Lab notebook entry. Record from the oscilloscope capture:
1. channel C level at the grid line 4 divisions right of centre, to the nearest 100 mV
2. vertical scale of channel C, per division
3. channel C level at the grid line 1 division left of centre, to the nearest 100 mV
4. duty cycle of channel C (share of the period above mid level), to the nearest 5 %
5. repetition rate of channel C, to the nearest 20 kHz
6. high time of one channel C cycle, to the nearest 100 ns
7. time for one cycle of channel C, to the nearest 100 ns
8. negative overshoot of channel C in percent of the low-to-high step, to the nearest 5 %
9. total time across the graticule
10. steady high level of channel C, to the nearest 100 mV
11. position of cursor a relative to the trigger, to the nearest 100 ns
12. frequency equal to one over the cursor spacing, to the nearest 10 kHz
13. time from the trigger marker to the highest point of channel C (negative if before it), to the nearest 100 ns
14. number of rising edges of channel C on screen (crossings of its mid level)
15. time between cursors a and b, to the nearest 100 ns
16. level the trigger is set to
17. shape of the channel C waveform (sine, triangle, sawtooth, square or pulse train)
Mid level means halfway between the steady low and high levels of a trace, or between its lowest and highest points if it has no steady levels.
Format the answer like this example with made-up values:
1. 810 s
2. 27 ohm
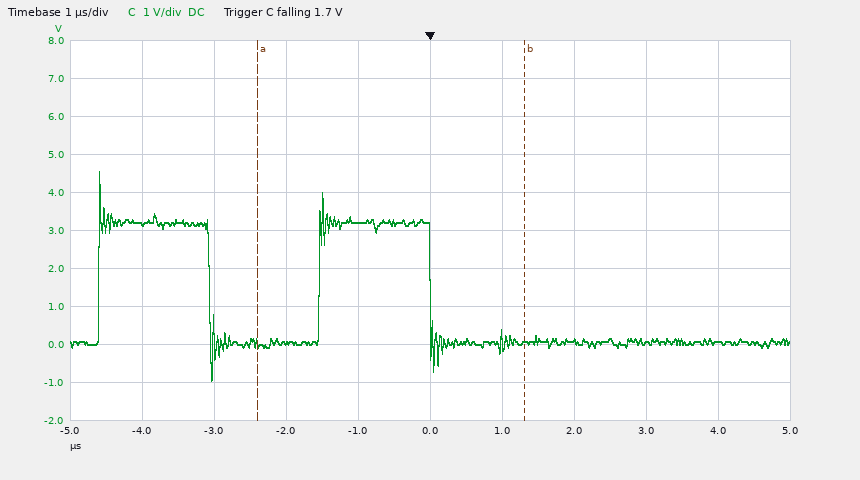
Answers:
1. 100 mV
2. 1 V
3. 3.2 V
4. 50 %
5. 320 kHz
6. 1.5 µs
7. 3.1 µs
8. 30 %
9. 10 µs
10. 3.2 V
11. -2.4 µs
12. 270 kHz
13. -4.6 µs
14. 2
15. 3.7 µs
16. 1.7 V
17. square
